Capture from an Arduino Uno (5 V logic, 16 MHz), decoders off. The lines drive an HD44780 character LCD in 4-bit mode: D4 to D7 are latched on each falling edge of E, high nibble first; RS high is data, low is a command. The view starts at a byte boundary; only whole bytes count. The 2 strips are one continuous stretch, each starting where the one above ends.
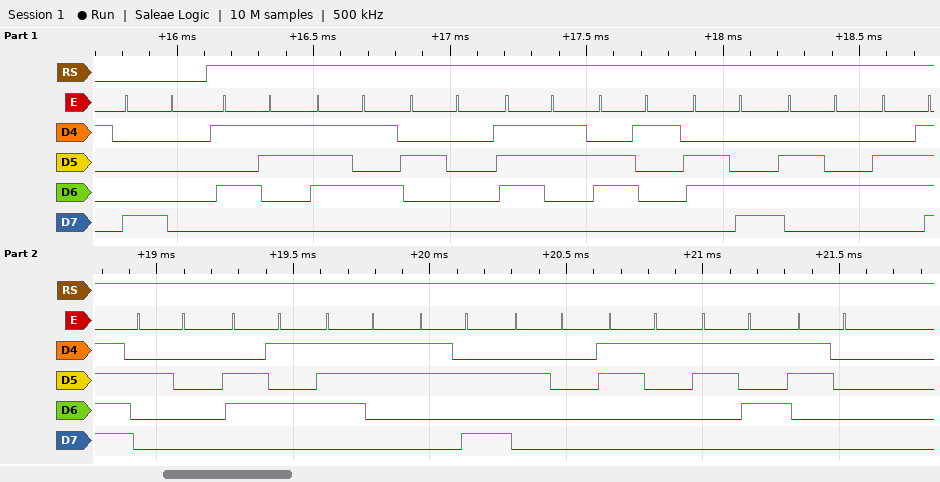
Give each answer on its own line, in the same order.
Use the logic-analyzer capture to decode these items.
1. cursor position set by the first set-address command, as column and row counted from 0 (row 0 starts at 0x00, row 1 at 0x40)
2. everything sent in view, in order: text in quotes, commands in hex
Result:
column 0, row 0
0x80 "Su saldo es: 150"
